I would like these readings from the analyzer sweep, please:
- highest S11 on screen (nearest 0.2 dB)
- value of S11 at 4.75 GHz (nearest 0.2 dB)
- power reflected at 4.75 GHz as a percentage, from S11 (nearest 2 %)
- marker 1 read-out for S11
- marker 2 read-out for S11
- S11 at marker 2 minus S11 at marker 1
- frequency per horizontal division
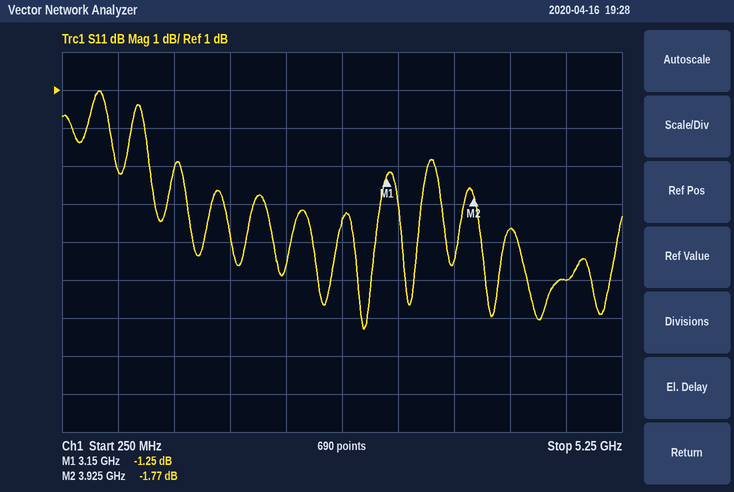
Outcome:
1.0 dB
-4.0 dB
40 %
-1.25 dB
-1.77 dB
-0.52 dB
500 MHz
